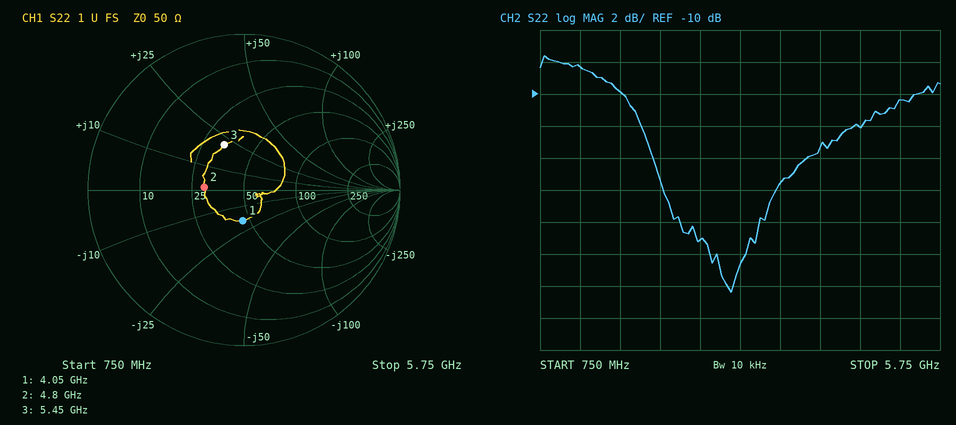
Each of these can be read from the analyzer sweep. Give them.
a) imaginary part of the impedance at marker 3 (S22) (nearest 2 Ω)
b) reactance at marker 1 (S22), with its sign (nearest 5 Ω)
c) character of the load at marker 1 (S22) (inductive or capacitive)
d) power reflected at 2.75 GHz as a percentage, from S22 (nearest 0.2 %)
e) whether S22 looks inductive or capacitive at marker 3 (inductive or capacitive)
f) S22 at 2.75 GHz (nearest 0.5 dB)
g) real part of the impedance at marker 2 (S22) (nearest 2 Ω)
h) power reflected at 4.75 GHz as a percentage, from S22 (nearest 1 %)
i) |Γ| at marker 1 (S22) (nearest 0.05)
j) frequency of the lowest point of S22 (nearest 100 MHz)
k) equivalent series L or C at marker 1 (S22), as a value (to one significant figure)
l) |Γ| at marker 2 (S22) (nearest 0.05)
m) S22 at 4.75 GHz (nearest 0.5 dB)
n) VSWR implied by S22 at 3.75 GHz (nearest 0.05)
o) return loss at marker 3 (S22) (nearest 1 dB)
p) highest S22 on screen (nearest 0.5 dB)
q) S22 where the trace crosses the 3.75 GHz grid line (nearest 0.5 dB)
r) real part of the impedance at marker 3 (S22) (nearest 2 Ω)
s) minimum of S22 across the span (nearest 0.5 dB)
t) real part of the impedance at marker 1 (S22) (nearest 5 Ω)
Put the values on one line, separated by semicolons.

+22 Ω; -20 Ω; capacitive; 1.2 %; inductive; -19.0 dB; 30 Ω; 6 %; 0.20; 3.1 GHz; 2 pF; 0.25; -12.0 dB; 1.40; 10 dB; -7.5 dB; -15.5 dB; 34 Ω; -22.5 dB; 45 Ω
